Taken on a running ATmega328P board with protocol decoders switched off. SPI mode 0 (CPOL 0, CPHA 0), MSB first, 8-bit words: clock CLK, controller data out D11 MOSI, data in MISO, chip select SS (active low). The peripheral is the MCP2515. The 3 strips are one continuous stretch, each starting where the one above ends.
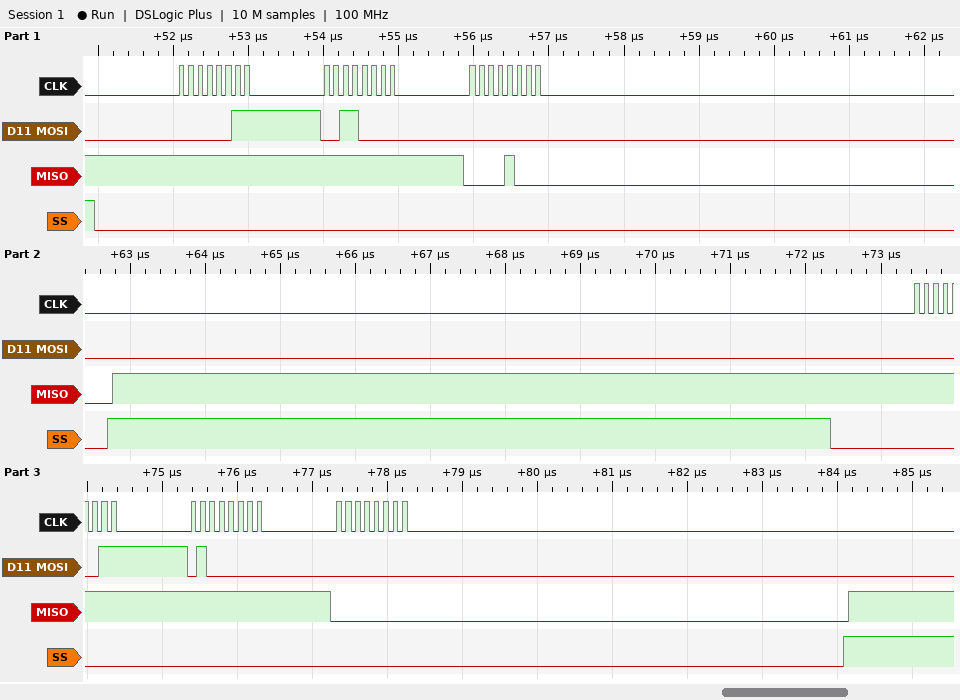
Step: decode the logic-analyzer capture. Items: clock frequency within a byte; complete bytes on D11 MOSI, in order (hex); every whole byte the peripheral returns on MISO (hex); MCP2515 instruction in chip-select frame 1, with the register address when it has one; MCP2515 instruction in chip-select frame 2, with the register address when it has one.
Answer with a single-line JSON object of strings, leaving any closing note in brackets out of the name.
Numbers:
{"clock frequency within a byte": "8 MHz", "complete bytes on D11 MOSI, in order": "03 30 00 03 40 00", "every whole byte the peripheral returns on MISO": "FF FF 08 FF FF 00", "MCP2515 instruction in chip-select frame 1, with the register address when it has one": "READ 0x30", "MCP2515 instruction in chip-select frame 2, with the register address when it has one": "READ 0x40"}
